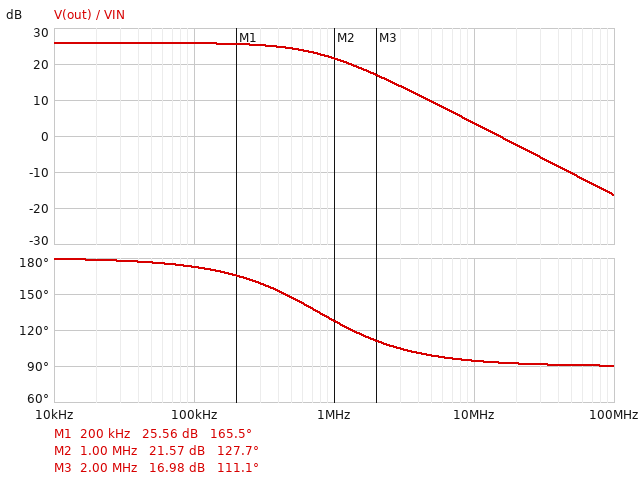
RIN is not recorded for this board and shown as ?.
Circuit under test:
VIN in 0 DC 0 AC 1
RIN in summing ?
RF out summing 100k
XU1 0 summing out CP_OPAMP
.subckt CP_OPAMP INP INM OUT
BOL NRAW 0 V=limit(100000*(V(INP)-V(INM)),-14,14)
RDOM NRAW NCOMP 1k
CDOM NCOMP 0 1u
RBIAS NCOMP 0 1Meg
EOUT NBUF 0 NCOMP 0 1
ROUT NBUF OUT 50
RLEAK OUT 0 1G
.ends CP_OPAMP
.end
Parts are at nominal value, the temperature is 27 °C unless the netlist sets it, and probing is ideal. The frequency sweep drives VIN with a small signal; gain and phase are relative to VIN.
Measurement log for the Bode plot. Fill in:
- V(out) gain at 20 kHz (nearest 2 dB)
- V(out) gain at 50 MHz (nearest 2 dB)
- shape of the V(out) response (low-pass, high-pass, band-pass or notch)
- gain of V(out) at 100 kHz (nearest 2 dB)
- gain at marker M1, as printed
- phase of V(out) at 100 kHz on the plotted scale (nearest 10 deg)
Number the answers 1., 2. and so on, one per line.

1. 26 dB
2. -10 dB
3. low-pass
4. 26 dB
5. 25.56 dB
6. 170 deg
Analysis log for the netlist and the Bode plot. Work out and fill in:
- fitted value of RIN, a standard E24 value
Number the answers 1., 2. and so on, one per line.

1. 5.1 kΩ
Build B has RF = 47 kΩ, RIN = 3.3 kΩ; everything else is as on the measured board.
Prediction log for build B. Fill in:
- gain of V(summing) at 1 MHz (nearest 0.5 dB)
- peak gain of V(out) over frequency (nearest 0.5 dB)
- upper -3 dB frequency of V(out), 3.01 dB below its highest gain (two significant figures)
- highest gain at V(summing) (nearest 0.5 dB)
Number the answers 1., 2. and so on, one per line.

1. -4.0 dB
2. 23.0 dB
3. 1.0 MHz
4. -0.5 dB
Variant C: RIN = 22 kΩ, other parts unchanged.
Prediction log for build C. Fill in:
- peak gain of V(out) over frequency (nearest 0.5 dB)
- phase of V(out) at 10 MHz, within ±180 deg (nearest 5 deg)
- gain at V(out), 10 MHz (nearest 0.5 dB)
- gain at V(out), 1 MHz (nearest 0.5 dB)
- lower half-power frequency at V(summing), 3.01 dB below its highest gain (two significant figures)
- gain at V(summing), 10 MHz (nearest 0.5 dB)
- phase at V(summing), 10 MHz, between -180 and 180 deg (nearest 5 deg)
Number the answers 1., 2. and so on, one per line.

1. 13.0 dB
2. 105 deg
3. 2.0 dB
4. 12.5 dB
5. 2.9 MHz
6. -2.0 dB
7. 15 deg
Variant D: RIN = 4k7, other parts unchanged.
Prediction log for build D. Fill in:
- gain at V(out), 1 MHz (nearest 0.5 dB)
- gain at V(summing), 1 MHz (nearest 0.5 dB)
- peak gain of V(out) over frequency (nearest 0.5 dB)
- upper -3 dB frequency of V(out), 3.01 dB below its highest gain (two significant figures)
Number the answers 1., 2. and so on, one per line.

1. 22.0 dB
2. -2.0 dB
3. 26.5 dB
4. 710 kHz
